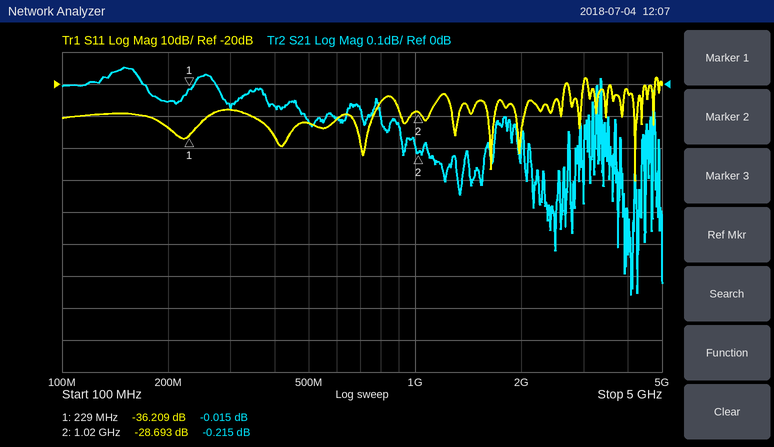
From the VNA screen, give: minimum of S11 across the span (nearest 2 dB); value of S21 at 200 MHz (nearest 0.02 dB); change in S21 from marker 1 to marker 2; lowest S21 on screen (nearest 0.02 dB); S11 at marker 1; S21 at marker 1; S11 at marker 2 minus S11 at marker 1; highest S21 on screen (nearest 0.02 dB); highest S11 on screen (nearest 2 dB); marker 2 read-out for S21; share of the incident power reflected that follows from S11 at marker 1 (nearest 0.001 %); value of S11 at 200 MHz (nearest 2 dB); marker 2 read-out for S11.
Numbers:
-50 dB
-0.06 dB
-0.200 dB
-0.66 dB
-36.209 dB
-0.015 dB
7.516 dB
0.06 dB
-18 dB
-0.215 dB
0.024 %
-34 dB
-28.693 dB
